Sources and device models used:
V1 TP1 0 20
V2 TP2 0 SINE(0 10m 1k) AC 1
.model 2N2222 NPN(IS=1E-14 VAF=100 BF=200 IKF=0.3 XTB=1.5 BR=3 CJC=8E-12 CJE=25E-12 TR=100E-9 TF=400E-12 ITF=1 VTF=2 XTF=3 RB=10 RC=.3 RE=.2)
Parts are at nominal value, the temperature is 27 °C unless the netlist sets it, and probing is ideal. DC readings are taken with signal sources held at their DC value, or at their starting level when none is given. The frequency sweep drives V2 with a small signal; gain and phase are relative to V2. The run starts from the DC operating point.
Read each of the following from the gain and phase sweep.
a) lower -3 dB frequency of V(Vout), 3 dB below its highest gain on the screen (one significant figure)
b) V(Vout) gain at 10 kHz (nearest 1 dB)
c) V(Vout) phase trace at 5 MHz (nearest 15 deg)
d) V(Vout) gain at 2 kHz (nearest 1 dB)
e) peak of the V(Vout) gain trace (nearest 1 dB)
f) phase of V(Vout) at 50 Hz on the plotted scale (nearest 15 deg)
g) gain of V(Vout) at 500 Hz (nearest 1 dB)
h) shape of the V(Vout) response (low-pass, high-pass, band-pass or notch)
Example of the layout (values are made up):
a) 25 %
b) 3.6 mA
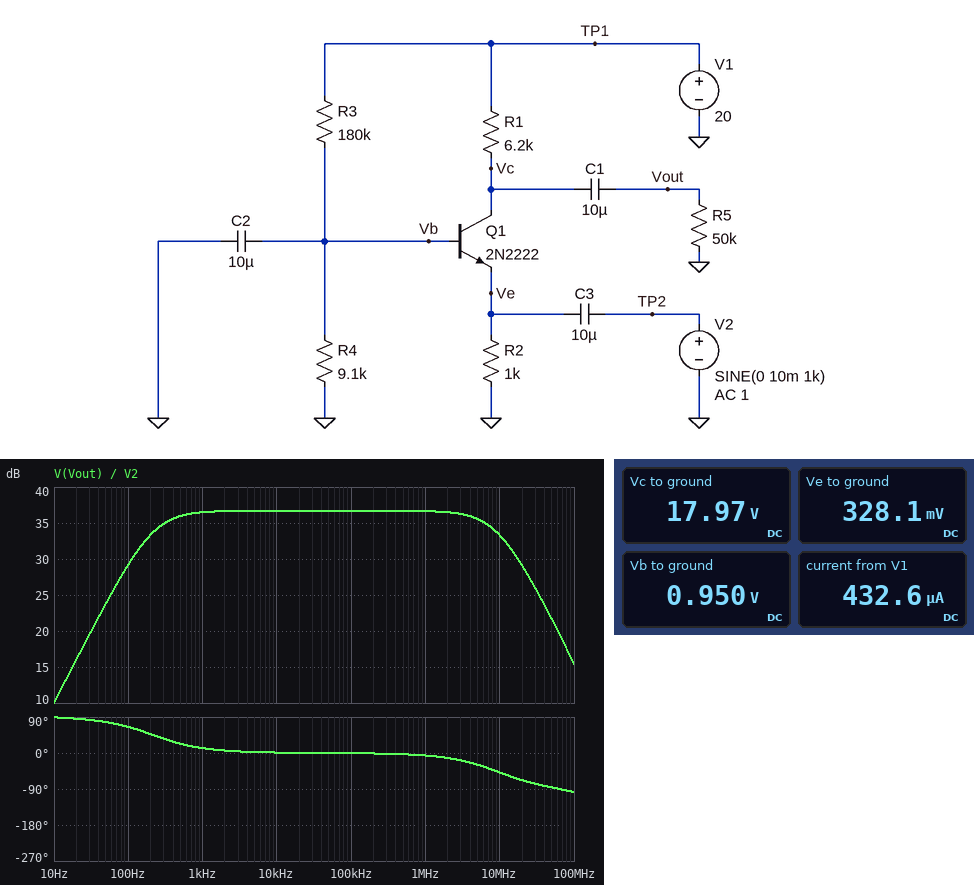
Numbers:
a) 200 Hz
b) 37 dB
c) -30 deg
d) 37 dB
e) 37 dB
f) 75 deg
g) 36 dB
h) band-pass
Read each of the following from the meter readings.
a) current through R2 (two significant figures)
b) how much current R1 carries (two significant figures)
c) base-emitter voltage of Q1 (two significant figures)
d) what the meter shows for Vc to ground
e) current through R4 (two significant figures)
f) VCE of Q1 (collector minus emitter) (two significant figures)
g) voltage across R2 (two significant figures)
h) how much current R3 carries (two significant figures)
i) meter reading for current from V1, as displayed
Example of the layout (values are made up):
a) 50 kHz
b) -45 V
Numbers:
a) 330 µA
b) 330 µA
c) 620 mV
d) 17.97 V
e) 100 µA
f) 18 V
g) 330 mV
h) 110 µA
i) 432.6 µA
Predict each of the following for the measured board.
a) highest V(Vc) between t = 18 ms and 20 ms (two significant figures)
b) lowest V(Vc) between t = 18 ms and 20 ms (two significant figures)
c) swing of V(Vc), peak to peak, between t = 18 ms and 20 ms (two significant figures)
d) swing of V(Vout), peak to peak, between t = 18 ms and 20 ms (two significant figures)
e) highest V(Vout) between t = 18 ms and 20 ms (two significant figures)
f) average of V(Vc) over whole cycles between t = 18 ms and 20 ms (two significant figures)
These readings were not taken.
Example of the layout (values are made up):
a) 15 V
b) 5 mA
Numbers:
a) 19 V
b) 17 V
c) 1.3 V
d) 1.3 V
e) 600 mV
f) 18 V
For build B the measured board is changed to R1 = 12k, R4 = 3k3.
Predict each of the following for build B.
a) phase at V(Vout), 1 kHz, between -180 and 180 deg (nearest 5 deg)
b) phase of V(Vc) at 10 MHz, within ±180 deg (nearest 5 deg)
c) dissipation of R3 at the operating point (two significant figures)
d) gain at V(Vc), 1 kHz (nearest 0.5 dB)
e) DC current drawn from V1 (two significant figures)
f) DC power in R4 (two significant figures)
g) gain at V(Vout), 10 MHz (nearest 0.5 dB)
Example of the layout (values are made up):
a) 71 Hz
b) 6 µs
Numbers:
a) 0 deg
b) 120 deg
c) 2.1 mW
d) -46.0 dB
e) 110 µA
f) 39 µW
g) -37.0 dB
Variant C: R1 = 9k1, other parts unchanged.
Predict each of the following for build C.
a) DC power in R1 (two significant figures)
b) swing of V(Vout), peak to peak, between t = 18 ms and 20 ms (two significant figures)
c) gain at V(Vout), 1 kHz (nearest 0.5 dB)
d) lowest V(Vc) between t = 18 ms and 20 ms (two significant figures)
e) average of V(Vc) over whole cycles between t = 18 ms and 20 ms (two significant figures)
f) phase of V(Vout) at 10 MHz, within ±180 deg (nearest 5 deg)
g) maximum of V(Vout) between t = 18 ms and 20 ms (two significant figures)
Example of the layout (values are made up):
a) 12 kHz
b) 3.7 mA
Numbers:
a) 970 µW
b) 1.8 V
c) 39.5 dB
d) 16 V
e) 17 V
f) -60 deg
g) 830 mV
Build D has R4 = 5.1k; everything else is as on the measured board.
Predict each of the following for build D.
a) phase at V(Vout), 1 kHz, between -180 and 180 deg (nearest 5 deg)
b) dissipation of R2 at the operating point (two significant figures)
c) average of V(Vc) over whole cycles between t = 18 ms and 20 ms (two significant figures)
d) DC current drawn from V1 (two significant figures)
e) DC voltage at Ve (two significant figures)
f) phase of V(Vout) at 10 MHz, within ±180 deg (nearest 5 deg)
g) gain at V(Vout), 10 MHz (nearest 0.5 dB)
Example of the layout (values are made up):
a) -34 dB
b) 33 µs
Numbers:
a) 0 deg
b) 170 nW
c) 20 V
d) 120 µA
e) 13 mV
f) -45 deg
g) 6.0 dB
